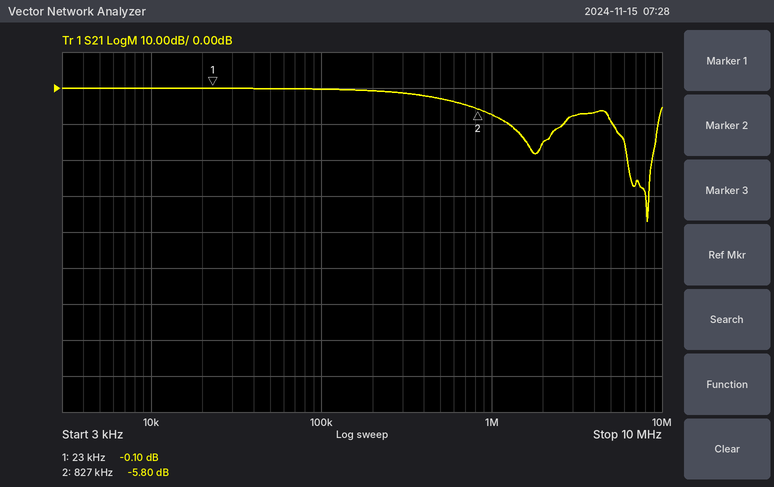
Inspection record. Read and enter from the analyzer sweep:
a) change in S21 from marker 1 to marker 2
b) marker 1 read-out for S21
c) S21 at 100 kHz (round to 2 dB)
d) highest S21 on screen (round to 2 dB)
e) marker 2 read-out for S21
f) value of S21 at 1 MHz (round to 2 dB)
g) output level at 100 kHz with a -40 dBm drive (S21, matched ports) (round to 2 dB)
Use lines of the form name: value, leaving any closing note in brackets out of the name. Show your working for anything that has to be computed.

change in S21 from marker 1 to marker 2: -5.8 − (-0.1) = -5.70 dB
marker 1 read-out for S21: -0.10 dB
S21 at 100 kHz: 0 dB
highest S21 on screen: 0 dB
marker 2 read-out for S21: -5.80 dB
value of S21 at 1 MHz: -8 dB
output level at 100 kHz with a -40 dBm drive (S21, matched ports): -40 dBm + (0 dB) = -40 dBm
